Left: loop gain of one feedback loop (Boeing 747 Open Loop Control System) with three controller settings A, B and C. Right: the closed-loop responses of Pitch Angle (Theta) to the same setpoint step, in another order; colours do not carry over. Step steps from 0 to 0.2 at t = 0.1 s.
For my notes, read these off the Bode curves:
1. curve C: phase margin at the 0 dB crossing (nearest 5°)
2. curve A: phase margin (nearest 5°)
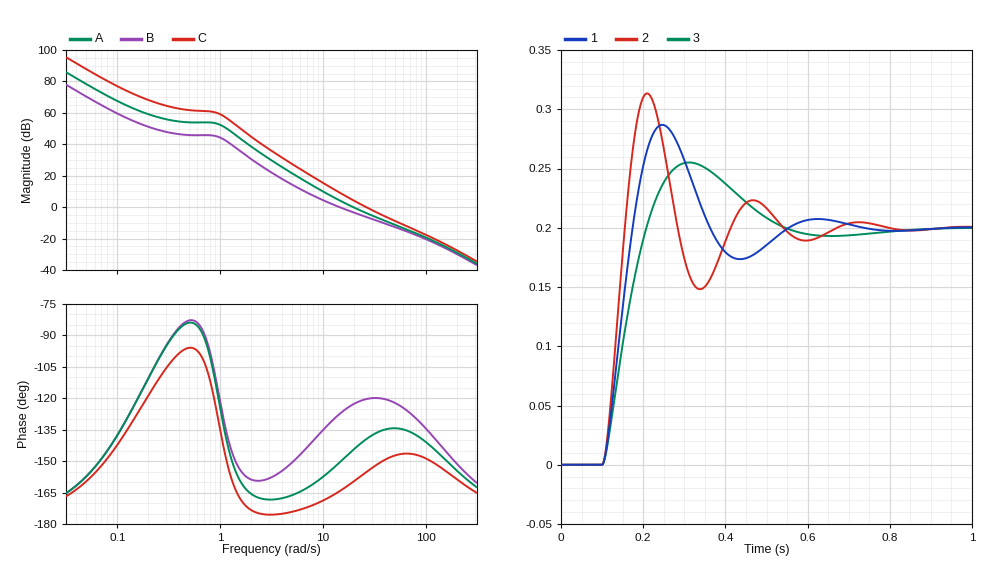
25°
35°
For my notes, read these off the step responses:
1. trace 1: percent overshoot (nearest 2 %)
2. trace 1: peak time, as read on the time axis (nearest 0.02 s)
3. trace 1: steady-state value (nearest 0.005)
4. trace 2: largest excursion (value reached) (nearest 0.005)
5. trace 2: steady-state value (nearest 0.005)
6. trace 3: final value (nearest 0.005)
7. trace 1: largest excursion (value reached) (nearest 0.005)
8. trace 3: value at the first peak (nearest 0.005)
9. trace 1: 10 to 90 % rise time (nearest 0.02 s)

44 %
0.24 s
0.200
0.315
0.200
0.200
0.285
0.255
0.06 s
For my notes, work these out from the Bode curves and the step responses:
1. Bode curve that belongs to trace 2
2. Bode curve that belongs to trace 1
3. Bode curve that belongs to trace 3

C
A
B
